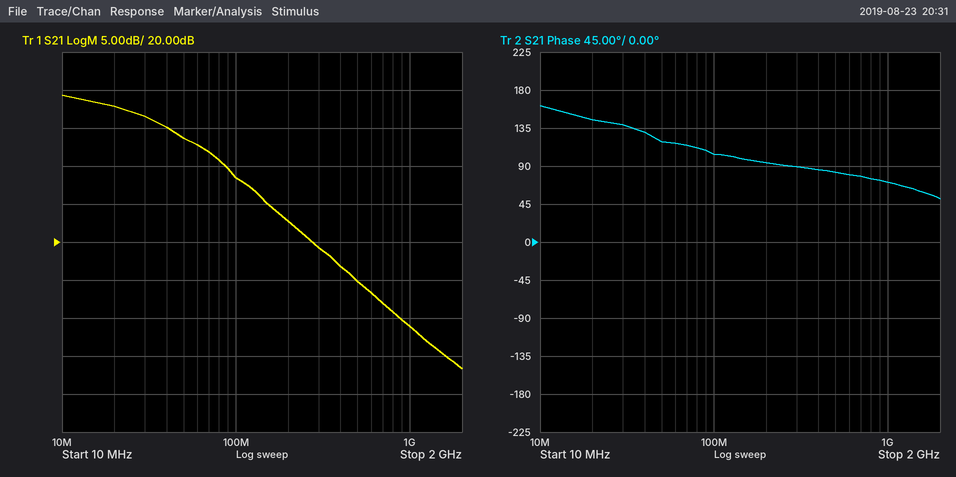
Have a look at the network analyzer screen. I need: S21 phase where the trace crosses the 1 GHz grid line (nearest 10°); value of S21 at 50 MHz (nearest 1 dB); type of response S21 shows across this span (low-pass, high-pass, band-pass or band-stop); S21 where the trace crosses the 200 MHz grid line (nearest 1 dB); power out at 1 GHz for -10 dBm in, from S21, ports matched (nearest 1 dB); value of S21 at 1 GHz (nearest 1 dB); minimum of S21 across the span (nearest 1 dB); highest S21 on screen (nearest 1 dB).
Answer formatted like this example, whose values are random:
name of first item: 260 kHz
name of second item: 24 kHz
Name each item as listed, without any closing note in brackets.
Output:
S21 phase where the trace crosses the 1 GHz grid line: 70°
value of S21 at 50 MHz: 34 dB
type of response S21 shows across this span: low-pass
S21 where the trace crosses the 200 MHz grid line: 23 dB
power out at 1 GHz for -10 dBm in, from S21, ports matched: -1 dBm
value of S21 at 1 GHz: 9 dB
minimum of S21 across the span: 3 dB
highest S21 on screen: 39 dB
